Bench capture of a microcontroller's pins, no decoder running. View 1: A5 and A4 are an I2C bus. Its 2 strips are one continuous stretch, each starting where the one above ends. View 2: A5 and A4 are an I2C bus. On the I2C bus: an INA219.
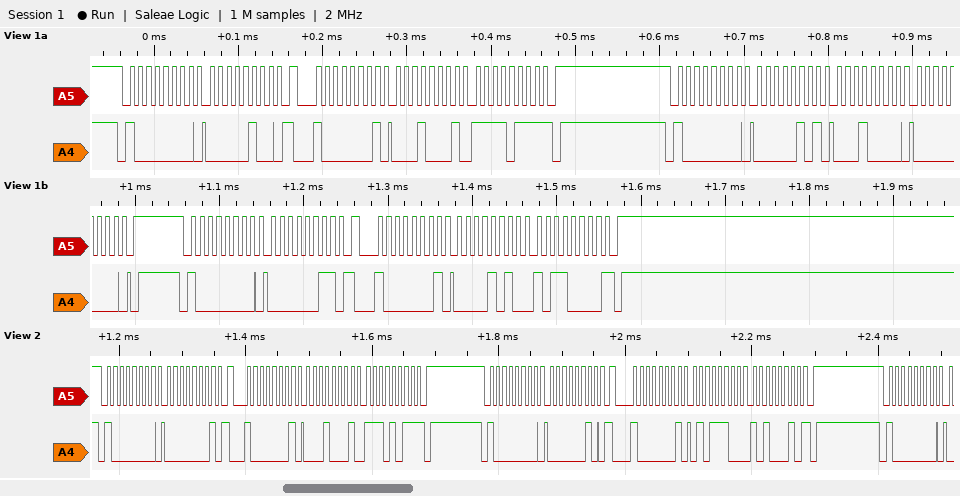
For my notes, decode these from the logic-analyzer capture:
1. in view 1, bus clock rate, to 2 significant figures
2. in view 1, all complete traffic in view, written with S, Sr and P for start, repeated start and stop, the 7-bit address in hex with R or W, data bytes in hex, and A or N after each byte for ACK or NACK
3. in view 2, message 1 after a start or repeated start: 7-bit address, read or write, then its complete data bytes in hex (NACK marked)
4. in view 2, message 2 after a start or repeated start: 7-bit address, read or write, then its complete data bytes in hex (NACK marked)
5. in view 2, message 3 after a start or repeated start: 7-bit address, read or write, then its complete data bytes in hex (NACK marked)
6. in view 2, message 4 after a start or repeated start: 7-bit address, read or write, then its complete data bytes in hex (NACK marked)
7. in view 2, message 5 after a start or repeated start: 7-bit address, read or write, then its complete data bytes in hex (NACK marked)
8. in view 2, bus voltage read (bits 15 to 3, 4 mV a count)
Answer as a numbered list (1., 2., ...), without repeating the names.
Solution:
1. 100 kHz
2. S 40W A 04 A Sr 40R A 11 A F7 N P S 40W A 05 A 10 A 00 A P S 40W A 03 A Sr 40R A 0A A B0 N P
3. 0x40 write: 01
4. 0x40 read: 11 EB NACK
5. 0x40 write: 02
6. 0x40 read: 5C A2 NACK
7. 0x40 write
8. 11.856 V
